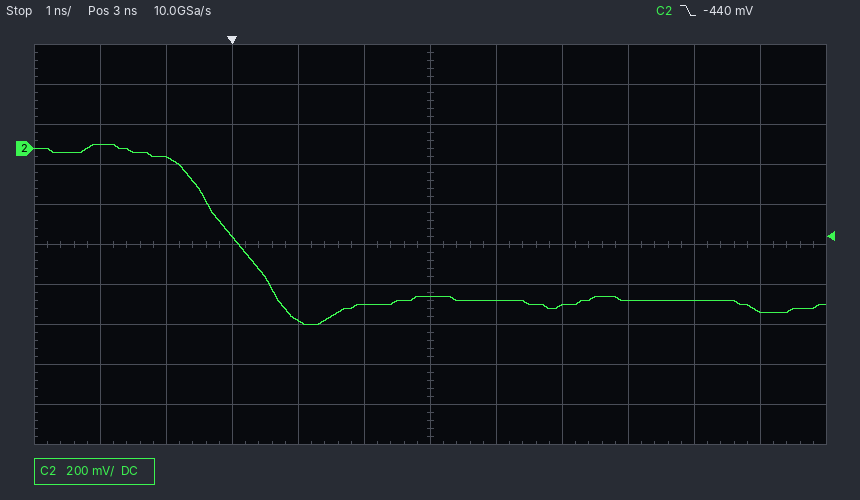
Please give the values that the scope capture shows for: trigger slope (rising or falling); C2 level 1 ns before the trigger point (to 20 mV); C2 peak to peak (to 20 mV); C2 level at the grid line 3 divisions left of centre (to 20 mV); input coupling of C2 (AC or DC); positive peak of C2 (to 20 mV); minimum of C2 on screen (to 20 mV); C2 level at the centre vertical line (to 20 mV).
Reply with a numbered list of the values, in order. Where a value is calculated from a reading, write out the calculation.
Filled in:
1. falling
2. -40 mV
3. 20 mV − (-880 mV) = 900 mV
4. -440 mV
5. DC
6. 20 mV
7. -880 mV
8. -740 mV
